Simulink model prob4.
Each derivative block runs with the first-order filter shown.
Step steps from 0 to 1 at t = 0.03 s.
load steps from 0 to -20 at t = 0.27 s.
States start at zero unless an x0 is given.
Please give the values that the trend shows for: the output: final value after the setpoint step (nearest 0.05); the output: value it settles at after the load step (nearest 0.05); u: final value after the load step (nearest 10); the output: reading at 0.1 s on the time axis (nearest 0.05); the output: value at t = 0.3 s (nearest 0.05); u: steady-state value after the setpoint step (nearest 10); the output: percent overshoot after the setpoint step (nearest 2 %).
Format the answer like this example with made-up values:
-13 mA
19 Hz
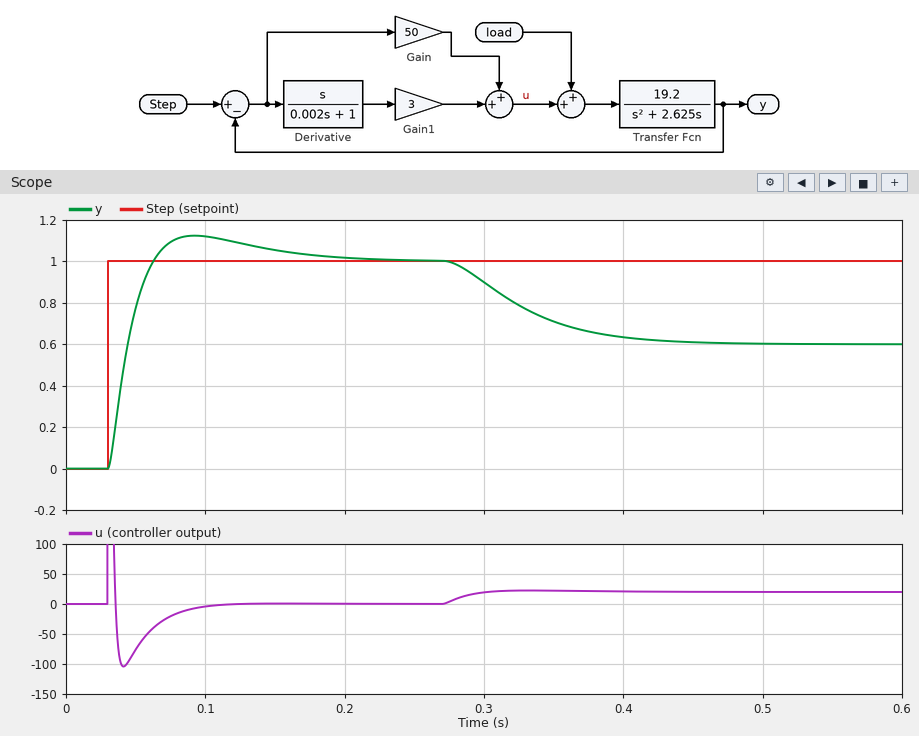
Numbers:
1.00
0.60
20
1.10
0.90
0
12 %
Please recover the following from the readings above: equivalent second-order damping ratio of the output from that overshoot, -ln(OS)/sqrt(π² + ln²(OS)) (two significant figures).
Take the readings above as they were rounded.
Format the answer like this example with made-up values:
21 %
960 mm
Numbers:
0.56
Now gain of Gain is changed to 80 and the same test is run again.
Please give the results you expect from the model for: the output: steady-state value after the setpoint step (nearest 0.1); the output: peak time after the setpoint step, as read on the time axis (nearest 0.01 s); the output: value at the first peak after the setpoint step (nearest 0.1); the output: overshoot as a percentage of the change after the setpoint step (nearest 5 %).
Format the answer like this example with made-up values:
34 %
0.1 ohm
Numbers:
1.0
0.08 s
1.2
20 %
